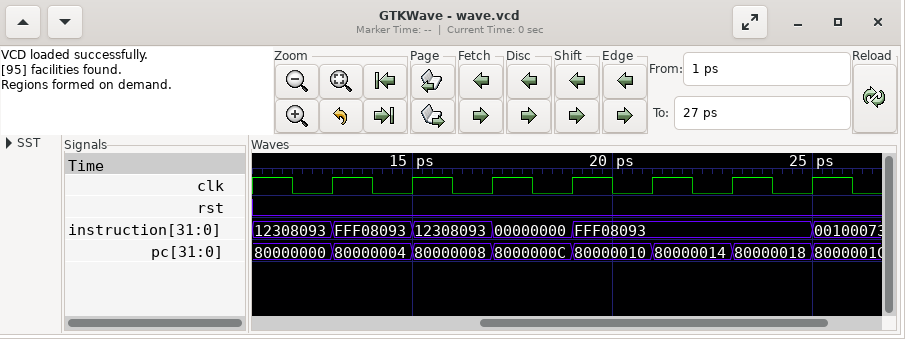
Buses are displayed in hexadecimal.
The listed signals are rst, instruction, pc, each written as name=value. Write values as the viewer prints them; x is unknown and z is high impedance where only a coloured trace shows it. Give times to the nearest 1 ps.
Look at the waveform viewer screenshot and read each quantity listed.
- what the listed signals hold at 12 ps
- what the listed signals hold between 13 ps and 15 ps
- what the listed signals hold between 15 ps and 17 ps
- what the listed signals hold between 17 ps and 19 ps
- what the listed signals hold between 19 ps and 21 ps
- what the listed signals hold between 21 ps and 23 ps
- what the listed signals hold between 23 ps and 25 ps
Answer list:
rst=0, instruction=12308093, pc=80000000
rst=0, instruction=FFF08093, pc=80000004
rst=0, instruction=12308093, pc=80000008
rst=0, instruction=00000000, pc=8000000C
rst=0, instruction=FFF08093, pc=80000010
rst=0, instruction=FFF08093, pc=80000014
rst=0, instruction=FFF08093, pc=80000018
